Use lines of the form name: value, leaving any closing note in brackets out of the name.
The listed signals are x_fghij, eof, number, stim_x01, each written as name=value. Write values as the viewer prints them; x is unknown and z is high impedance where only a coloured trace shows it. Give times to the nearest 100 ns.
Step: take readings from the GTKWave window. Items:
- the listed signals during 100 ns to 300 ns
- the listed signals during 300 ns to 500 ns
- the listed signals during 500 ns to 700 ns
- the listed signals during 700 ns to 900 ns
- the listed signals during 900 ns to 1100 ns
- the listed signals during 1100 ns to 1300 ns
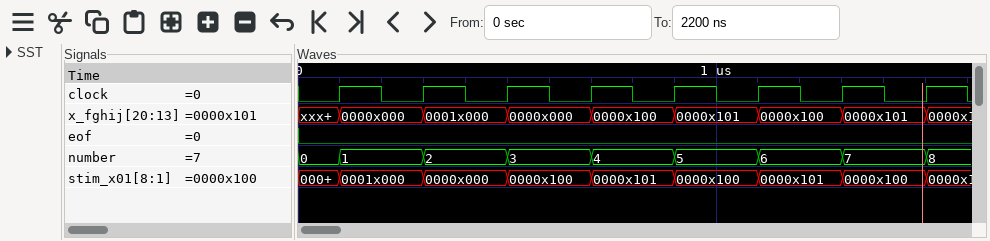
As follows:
the listed signals during 100 ns to 300 ns: x_fghij=0000x000, eof=0, number=1, stim_x01=0001x000
the listed signals during 300 ns to 500 ns: x_fghij=0001x000, eof=0, number=2, stim_x01=0000x000
the listed signals during 500 ns to 700 ns: x_fghij=0000x000, eof=0, number=3, stim_x01=0000x100
the listed signals during 700 ns to 900 ns: x_fghij=0000x100, eof=0, number=4, stim_x01=0000x101
the listed signals during 900 ns to 1100 ns: x_fghij=0000x101, eof=0, number=5, stim_x01=0000x100
the listed signals during 1100 ns to 1300 ns: x_fghij=0000x100, eof=0, number=6, stim_x01=0000x101
